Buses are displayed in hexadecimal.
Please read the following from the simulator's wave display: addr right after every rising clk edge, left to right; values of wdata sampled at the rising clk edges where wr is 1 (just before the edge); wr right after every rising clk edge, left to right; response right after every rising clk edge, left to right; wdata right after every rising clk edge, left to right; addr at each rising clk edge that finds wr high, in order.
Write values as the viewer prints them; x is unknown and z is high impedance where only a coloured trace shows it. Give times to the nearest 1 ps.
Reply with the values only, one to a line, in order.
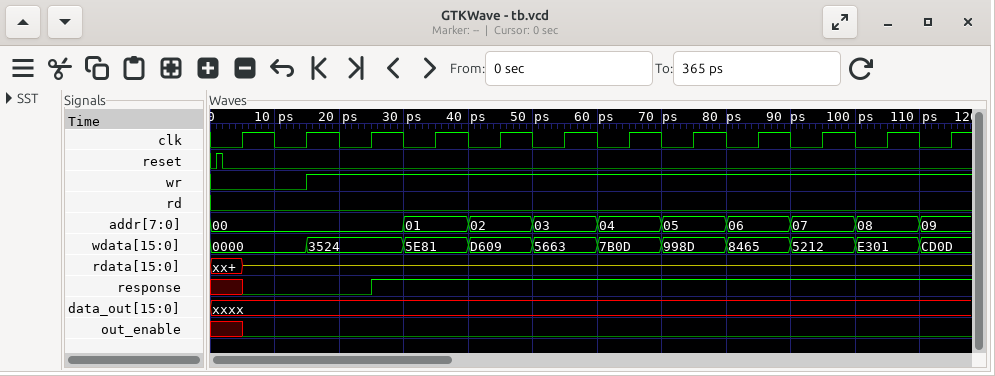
00, 00, 00, 01, 02, 03, 04, 05, 06, 07, 08, 09
3524, 5E81, D609, 5663, 7B0D, 998D, 8465, 5212, E301, CD0D
0 1 1 1 1 1 1 1 1 1 1 1
0 0 1 1 1 1 1 1 1 1 1 1
0000, 3524, 3524, 5E81, D609, 5663, 7B0D, 998D, 8465, 5212, E301, CD0D
00, 01, 02, 03, 04, 05, 06, 07, 08, 09
